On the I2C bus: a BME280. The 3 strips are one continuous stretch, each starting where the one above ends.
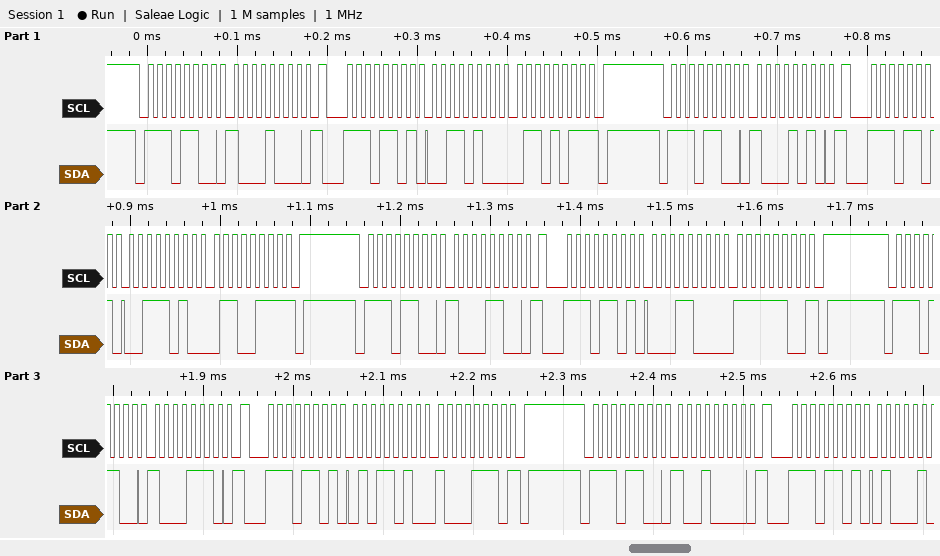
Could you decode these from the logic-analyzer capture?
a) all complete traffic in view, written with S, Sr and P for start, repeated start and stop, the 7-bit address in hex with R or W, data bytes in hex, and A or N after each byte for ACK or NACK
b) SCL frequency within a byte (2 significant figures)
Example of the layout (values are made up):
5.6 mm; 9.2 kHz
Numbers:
S 76W A 88 A Sr 76R A 34 A 6B N P S 76W A 8A A Sr 76R A 3A A 67 N P S 76W A 8C A Sr 76R A 18 A FC N P S 76W A 8E A Sr 76R A 5A A 8E N P S 76W A 90 A Sr 76R A; 100 kHz
